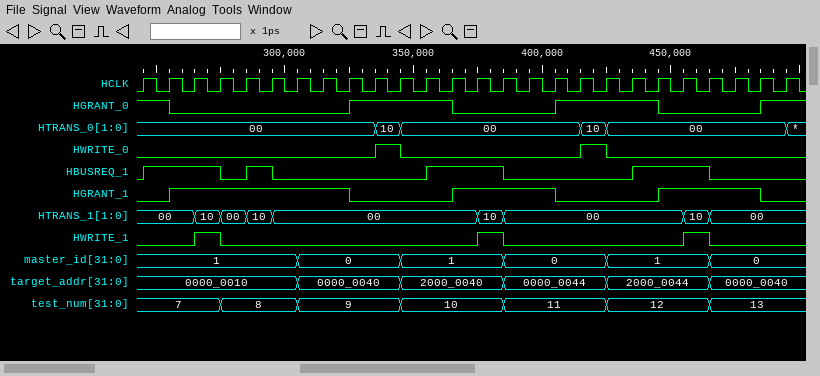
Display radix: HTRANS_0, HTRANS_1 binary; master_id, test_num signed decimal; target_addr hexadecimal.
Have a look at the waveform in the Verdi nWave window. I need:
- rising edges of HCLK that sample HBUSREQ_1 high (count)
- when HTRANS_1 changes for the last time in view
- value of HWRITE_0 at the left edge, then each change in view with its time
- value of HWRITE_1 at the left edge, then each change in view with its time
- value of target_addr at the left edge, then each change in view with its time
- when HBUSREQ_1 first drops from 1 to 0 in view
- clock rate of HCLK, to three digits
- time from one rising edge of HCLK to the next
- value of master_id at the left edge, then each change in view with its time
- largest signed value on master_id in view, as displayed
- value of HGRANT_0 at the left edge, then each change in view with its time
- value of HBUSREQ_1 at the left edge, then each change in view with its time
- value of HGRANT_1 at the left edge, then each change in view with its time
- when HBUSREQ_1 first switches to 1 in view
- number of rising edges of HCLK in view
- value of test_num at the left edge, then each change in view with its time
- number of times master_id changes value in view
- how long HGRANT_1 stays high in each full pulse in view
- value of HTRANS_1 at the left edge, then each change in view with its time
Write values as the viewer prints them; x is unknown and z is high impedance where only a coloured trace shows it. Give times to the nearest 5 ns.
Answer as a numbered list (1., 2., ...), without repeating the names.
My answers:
1. 10
2. 465 ns
3. 0, 1 at 335 ns, 0 at 345 ns, 1 at 415 ns, 0 at 425 ns
4. 0, 1 at 265 ns, 0 at 275 ns, 1 at 375 ns, 0 at 385 ns, 1 at 455 ns, 0 at 465 ns
5. 0000_0010, 0000_0040 at 305 ns, 2000_0040 at 345 ns, 0000_0044 at 385 ns, 2000_0044 at 425 ns, 0000_0040 at 465 ns
6. 275 ns
7. 100 MHz
8. 10 ns
9. 1, 0 at 305 ns, 1 at 345 ns, 0 at 385 ns, 1 at 425 ns, 0 at 465 ns
10. 1
11. 1, 0 at 255 ns, 1 at 325 ns, 0 at 365 ns, 1 at 405 ns, 0 at 445 ns, 1 at 485 ns
12. 0, 1 at 245 ns, 0 at 275 ns, 1 at 285 ns, 0 at 295 ns, 1 at 355 ns, 0 at 385 ns, 1 at 435 ns, 0 at 465 ns
13. 0, 1 at 255 ns, 0 at 325 ns, 1 at 365 ns, 0 at 405 ns, 1 at 445 ns, 0 at 485 ns
14. 245 ns
15. 26
16. 7, 8 at 275 ns, 9 at 305 ns, 10 at 345 ns, 11 at 385 ns, 12 at 425 ns, 13 at 465 ns
17. 5
18. 70 ns, 40 ns, 40 ns
19. 00, 10 at 265 ns, 00 at 275 ns, 10 at 285 ns, 00 at 295 ns, 10 at 375 ns, 00 at 385 ns, 10 at 455 ns, 00 at 465 ns
